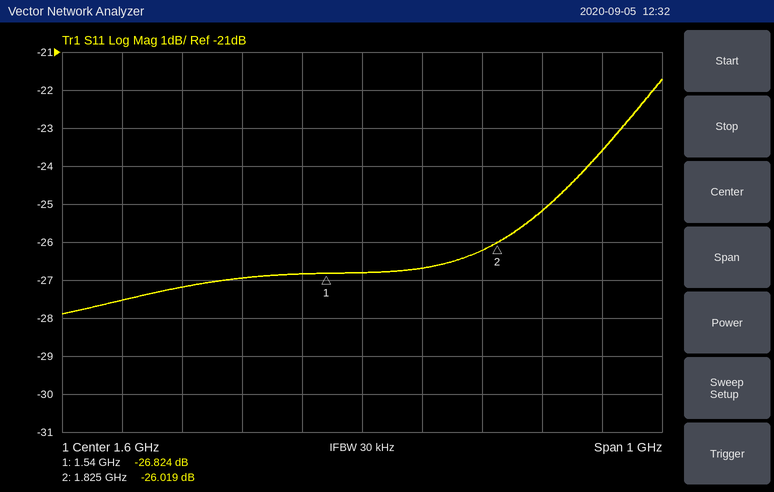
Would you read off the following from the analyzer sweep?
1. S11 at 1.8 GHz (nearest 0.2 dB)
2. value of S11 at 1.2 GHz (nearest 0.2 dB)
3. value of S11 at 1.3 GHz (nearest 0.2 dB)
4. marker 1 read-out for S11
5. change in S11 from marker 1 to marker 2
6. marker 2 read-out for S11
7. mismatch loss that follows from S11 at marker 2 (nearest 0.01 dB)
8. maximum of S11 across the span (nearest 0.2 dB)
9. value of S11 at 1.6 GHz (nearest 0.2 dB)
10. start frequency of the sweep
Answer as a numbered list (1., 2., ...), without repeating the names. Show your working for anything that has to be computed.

1. -26.2 dB
2. -27.6 dB
3. -27.2 dB
4. -26.824 dB
5. -26.019 − (-26.824) = 0.805 dB
6. -26.019 dB
7. −10 log10(1 − 10^(-26.019/10)) ≈ 0.01 dB
8. -21.8 dB
9. -26.8 dB
10. 1.1 GHz
